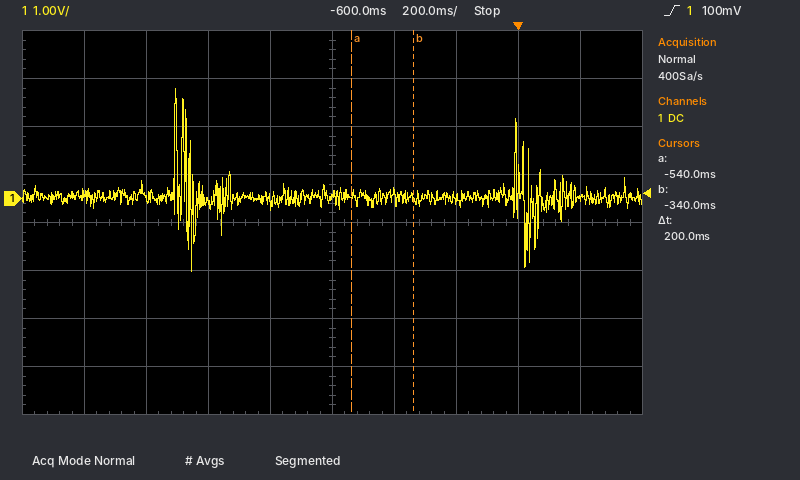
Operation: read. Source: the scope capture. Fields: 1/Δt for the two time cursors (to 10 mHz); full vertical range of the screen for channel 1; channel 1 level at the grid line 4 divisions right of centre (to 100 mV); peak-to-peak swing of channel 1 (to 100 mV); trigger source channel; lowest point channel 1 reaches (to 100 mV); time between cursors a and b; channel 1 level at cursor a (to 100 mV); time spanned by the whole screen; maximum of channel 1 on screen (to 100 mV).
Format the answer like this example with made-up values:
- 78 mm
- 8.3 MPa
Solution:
- 5.00 Hz
- 8 V
- 0.0 V
- 3.8 V
- channel 1
- -1.5 V
- 200 ms
- 100 mV
- 2 s
- 2.3 V
